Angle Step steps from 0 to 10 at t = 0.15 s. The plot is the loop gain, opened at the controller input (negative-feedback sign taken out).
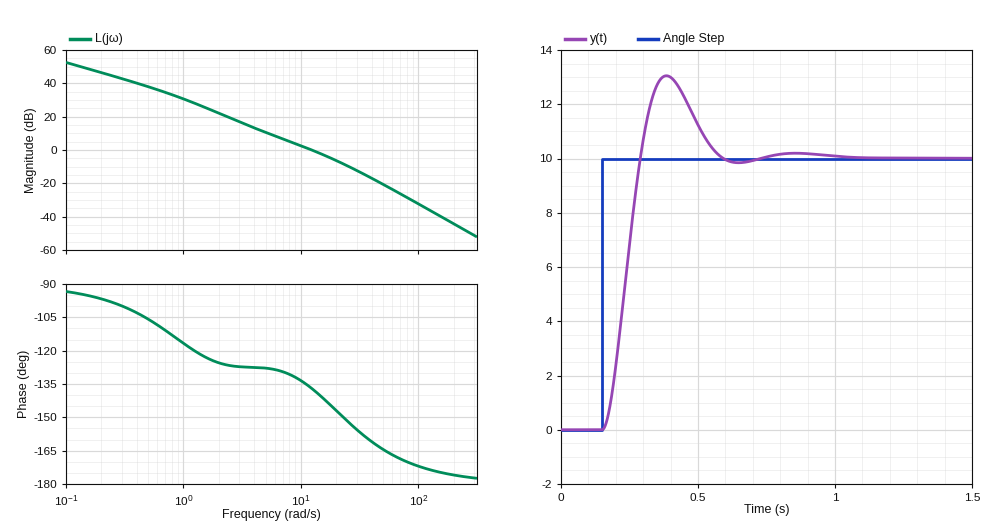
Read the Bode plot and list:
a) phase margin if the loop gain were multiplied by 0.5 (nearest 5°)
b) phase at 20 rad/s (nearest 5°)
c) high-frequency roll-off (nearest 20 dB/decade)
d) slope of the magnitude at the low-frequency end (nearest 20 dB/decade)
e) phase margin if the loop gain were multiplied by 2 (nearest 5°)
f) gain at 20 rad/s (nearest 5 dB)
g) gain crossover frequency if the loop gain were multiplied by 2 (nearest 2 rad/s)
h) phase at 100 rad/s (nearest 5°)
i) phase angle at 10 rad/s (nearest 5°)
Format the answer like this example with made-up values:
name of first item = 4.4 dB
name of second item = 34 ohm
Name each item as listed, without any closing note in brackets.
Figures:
phase margin if the loop gain were multiplied by 0.5 = 50°
phase at 20 rad/s = -145°
high-frequency roll-off = -40 dB/decade
slope of the magnitude at the low-frequency end = -20 dB/decade
phase margin if the loop gain were multiplied by 2 = 35°
gain at 20 rad/s = -5 dB
gain crossover frequency if the loop gain were multiplied by 2 = 20 rad/s
phase at 100 rad/s = -170°
phase angle at 10 rad/s = -135°
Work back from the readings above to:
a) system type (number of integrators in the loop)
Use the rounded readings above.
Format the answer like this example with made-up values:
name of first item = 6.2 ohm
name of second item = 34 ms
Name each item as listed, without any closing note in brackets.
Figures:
system type = 1
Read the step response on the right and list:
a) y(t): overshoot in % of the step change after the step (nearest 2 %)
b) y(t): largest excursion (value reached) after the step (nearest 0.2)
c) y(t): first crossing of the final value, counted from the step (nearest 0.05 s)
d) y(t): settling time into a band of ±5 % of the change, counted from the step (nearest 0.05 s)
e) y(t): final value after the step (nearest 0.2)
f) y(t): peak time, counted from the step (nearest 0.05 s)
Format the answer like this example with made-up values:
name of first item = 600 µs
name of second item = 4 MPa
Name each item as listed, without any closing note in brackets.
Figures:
y(t): overshoot in % of the step change after the step = 30 %
y(t): largest excursion (value reached) after the step = 13.0
y(t): first crossing of the final value, counted from the step = 0.15 s
y(t): settling time into a band of ±5 % of the change, counted from the step = 0.40 s
y(t): final value after the step = 10.0
y(t): peak time, counted from the step = 0.25 s
